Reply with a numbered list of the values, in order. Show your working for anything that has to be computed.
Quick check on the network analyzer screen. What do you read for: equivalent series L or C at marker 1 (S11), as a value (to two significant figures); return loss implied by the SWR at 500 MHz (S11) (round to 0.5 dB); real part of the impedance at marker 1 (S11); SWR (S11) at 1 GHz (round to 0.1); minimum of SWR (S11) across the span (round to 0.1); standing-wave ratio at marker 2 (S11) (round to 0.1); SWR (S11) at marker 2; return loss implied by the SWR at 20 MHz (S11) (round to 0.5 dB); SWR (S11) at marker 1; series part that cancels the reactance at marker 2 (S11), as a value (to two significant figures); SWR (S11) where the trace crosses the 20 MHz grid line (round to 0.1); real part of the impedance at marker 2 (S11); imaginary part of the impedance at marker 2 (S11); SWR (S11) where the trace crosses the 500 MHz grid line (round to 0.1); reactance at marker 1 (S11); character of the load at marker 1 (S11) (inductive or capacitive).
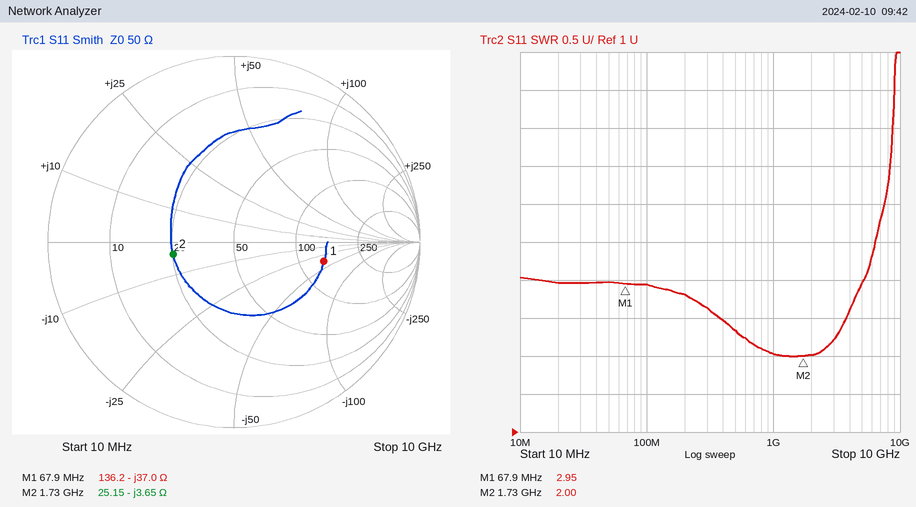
1. C = 1/(2π × 67.9 MHz × 37 Ω) ≈ 63 pF
2. −20 log10((2.3 − 1)/(2.3 + 1)) ≈ 8.09 dB, so 8.0 dB to the nearest 0.5 dB
3. 136.2 Ω
4. 2.0
5. 2.0
6. 2.0
7. 2.00
8. −20 log10((3 − 1)/(3 + 1)) ≈ 6.0 dB
9. 2.95
10. L = 3.65 Ω/(2π × 1.73 GHz) ≈ 336 pH, so 340 pH to two significant figures
11. 3.0
12. 25.15 Ω
13. -3.65 Ω
14. 2.3
15. -37.0 Ω
16. capacitive
